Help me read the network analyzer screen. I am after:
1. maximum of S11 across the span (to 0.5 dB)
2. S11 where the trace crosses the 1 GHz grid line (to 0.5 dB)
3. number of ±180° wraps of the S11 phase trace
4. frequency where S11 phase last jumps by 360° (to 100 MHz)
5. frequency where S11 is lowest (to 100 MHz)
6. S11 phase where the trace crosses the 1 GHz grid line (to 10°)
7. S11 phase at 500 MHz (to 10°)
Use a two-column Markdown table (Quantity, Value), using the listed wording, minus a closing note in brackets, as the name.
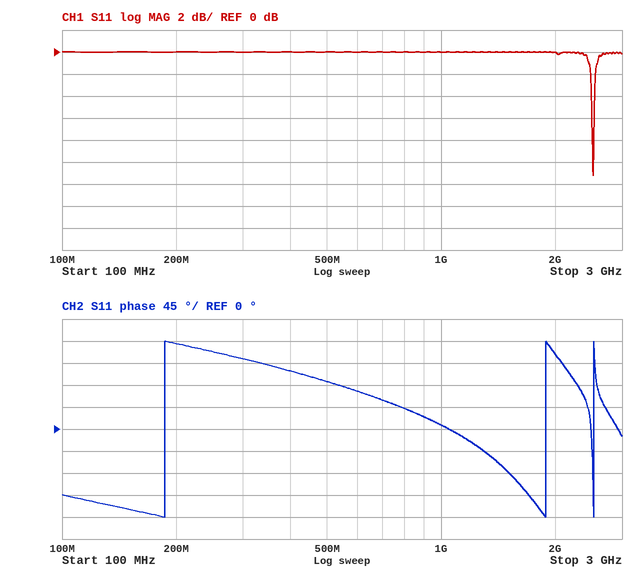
| Quantity | Value |
|---|---|
| maximum of S11 across the span | 0.0 dB |
| S11 where the trace crosses the 1 GHz grid line | 0.0 dB |
| number of ±180° wraps of the S11 phase trace | 3 |
| frequency where S11 phase last jumps by 360° | 2.5 GHz |
| frequency where S11 is lowest | 2.5 GHz |
| S11 phase where the trace crosses the 1 GHz grid line | 10° |
| S11 phase at 500 MHz | 100° |
